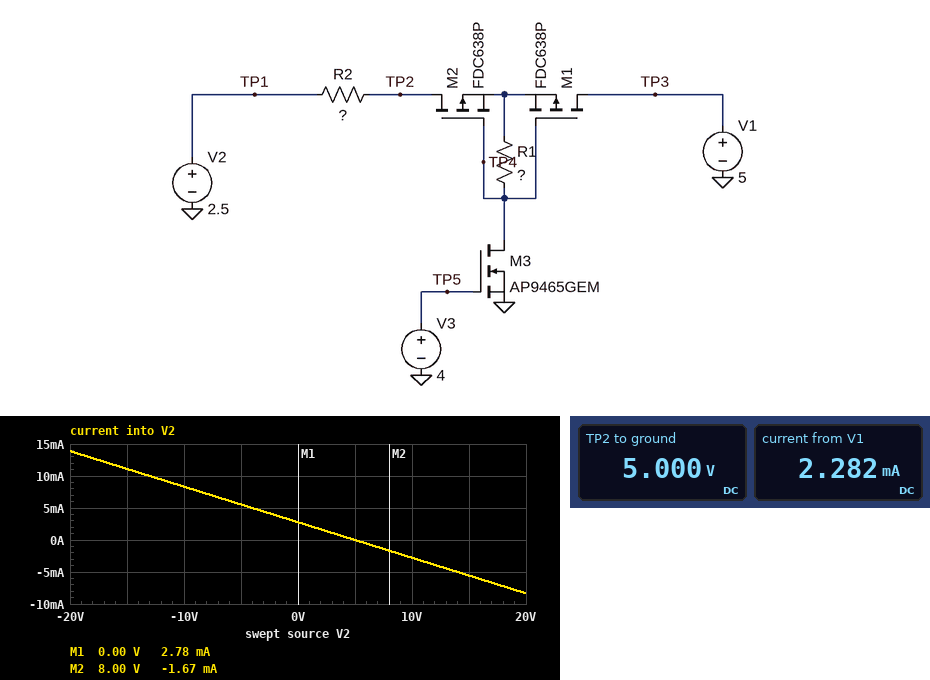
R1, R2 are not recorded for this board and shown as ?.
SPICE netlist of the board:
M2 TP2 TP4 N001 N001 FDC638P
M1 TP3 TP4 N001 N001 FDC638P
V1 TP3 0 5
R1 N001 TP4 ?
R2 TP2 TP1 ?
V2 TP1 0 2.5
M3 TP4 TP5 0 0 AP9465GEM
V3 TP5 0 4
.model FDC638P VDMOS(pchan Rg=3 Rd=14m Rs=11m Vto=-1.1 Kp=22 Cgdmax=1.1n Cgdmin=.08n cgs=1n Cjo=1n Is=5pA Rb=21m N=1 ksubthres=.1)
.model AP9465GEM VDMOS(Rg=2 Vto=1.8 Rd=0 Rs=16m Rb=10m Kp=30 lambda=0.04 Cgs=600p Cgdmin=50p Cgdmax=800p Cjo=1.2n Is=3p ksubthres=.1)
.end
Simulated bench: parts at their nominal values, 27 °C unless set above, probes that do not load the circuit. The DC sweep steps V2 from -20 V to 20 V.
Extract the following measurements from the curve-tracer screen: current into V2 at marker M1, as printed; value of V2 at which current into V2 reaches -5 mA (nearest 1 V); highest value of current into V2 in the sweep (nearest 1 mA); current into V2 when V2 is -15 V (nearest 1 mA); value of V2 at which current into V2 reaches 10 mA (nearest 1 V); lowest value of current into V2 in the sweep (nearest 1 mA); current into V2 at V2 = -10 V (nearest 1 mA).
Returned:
2.78 mA
14 V
14 mA
11 mA
-13 V
-8 mA
8 mA
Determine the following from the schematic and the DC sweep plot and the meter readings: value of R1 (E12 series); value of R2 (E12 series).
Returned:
5.6 kΩ
1.8 kΩ
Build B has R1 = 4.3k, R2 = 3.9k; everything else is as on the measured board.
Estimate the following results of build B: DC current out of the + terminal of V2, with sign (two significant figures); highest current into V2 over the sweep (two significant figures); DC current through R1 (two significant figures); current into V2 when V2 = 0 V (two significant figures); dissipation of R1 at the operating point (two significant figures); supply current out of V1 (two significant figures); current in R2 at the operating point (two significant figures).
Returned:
-640 µA
6.4 mA
1.2 mA
1.3 mA
5.8 mW
1.8 mA
640 µA
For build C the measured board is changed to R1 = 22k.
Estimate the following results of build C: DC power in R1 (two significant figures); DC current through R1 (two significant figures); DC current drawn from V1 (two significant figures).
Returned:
1.1 mW
230 µA
1.6 mA
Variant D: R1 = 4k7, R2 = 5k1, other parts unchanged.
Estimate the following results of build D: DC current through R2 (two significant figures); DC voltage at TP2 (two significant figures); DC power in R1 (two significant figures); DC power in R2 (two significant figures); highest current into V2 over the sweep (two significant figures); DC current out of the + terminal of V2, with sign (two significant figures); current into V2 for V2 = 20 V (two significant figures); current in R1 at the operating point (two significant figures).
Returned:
490 µA
5.0 V
5.3 mW
1.2 mW
4.9 mA
-490 µA
-2.9 mA
1.1 mA
